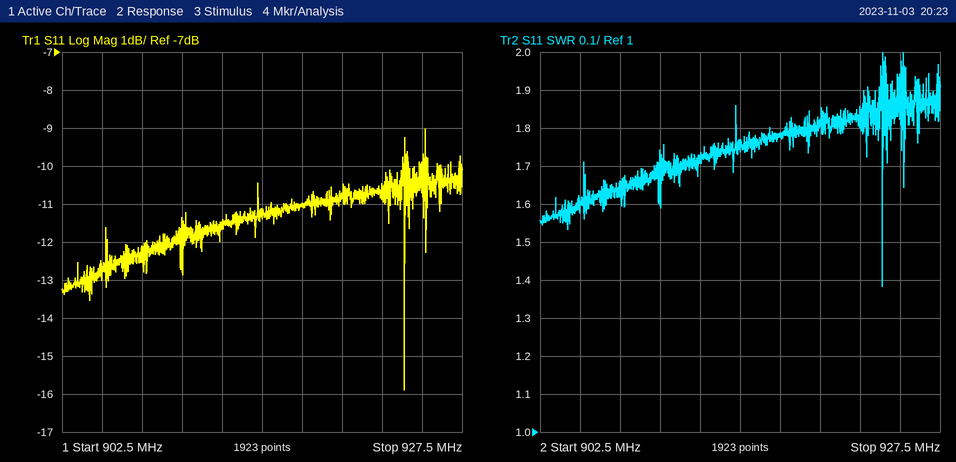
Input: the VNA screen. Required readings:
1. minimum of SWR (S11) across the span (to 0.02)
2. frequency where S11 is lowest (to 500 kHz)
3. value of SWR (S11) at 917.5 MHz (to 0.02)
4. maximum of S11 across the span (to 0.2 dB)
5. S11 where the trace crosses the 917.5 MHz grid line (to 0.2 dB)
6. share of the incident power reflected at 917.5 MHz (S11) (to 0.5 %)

1.38
924.0 MHz
1.78
-9.0 dB
-11.0 dB
8.0 %
